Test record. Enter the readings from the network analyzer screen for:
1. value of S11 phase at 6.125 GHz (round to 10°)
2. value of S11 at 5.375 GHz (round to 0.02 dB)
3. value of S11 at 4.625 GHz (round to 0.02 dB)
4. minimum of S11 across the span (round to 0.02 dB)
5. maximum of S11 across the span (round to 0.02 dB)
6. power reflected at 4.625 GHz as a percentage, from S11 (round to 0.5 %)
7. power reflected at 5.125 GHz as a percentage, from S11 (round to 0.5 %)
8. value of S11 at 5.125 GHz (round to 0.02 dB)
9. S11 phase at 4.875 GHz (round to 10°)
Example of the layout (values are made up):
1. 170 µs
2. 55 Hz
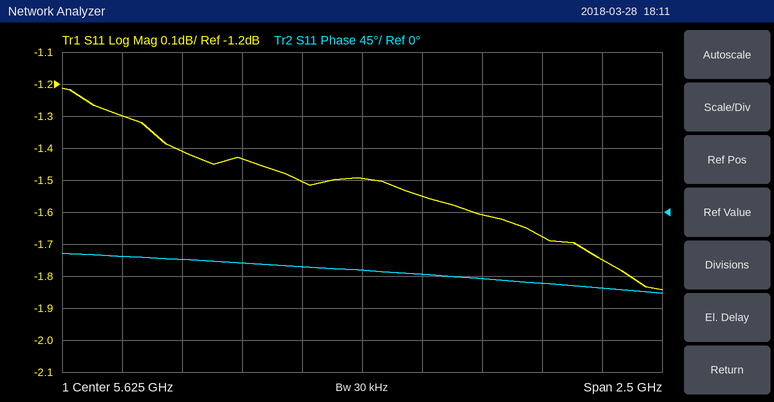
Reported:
1. -90°
2. -1.50 dB
3. -1.30 dB
4. -1.84 dB
5. -1.22 dB
6. 74.0 %
7. 72.0 %
8. -1.44 dB
9. -70°
